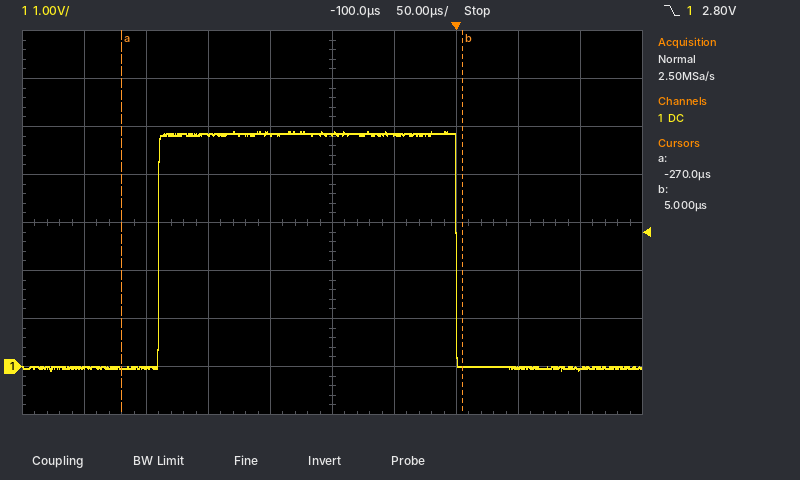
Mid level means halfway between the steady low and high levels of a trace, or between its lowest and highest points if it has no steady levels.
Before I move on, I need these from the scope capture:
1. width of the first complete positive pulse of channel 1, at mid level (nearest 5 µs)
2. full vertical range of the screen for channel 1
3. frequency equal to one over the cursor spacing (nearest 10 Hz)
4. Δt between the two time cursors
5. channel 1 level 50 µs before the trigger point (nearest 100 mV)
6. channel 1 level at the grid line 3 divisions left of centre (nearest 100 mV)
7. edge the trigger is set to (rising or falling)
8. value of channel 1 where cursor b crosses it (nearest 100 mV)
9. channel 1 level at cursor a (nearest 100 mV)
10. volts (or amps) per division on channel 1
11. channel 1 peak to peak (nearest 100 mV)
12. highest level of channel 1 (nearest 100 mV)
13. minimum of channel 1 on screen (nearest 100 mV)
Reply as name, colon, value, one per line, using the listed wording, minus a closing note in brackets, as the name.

width of the first complete positive pulse of channel 1, at mid level: 240 µs
full vertical range of the screen for channel 1: 8 V
frequency equal to one over the cursor spacing: 3.64 kHz
Δt between the two time cursors: 275 µs
channel 1 level 50 µs before the trigger point: 4.8 V
channel 1 level at the grid line 3 divisions left of centre: 0.0 V
edge the trigger is set to: falling
value of channel 1 where cursor b crosses it: 0.0 V
channel 1 level at cursor a: 0.0 V
volts (or amps) per division on channel 1: 1 V
channel 1 peak to peak: 5.0 V
highest level of channel 1: 4.9 V
minimum of channel 1 on screen: -100 mV
